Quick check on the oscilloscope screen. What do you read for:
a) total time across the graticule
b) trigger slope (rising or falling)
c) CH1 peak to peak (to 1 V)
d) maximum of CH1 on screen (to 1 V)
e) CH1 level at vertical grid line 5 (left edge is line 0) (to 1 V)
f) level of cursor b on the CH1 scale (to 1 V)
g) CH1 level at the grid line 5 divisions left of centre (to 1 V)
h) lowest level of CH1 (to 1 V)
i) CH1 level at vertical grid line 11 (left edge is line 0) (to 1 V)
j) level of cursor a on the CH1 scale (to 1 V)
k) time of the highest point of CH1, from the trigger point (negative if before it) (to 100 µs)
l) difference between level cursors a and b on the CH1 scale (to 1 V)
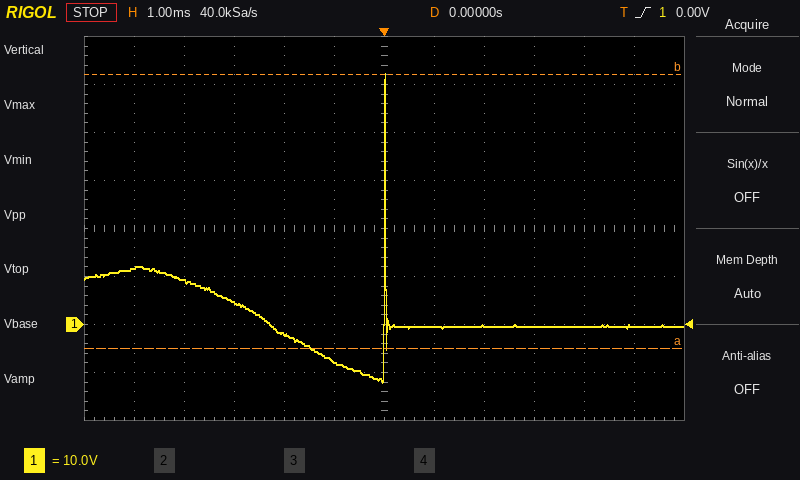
12 ms
rising
64 V
52 V
-8 V
52 V
12 V
-12 V
0 V
-5 V
0.0 ms
57 V
